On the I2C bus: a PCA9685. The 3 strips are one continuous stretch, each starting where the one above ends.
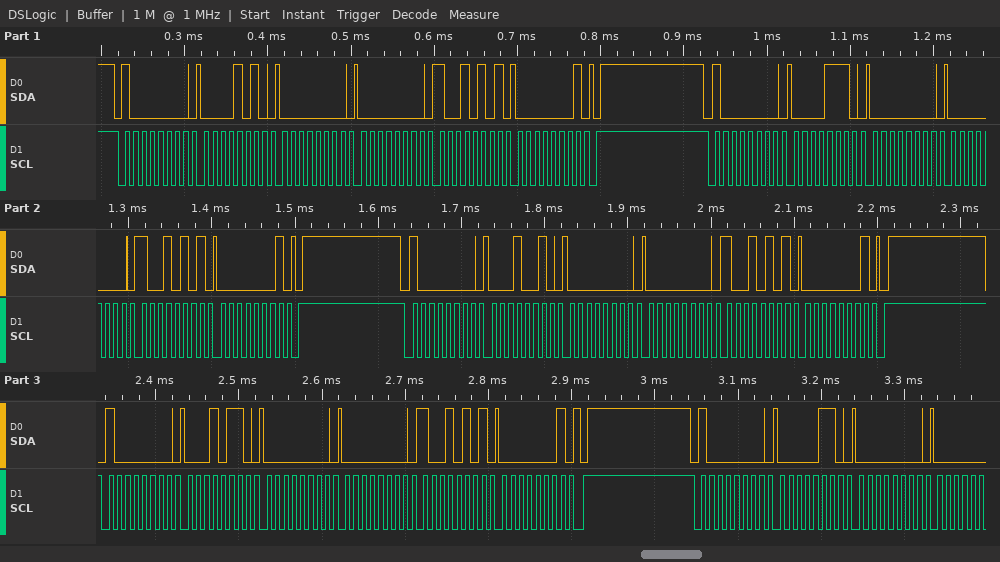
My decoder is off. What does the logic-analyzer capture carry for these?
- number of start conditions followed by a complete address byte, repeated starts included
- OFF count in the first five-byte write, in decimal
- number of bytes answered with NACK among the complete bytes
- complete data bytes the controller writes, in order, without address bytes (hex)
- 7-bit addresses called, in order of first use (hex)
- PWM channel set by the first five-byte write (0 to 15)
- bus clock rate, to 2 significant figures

5
405
0
0A 00 00 95 01 0E 00 00 95 01 12 00 00 95 01 16 00 00 95 01 06 00
0x40
1
100 kHz
